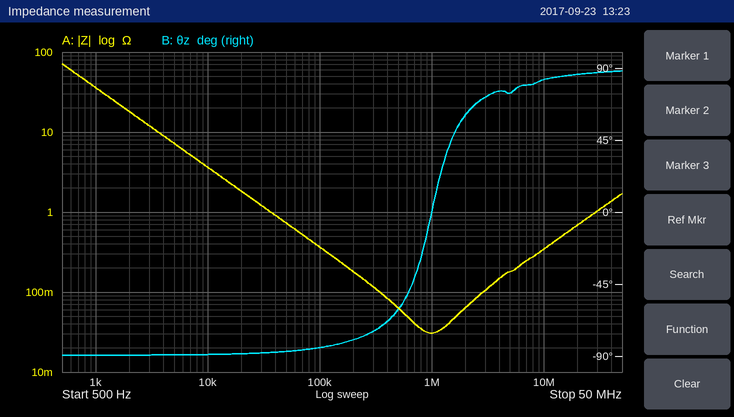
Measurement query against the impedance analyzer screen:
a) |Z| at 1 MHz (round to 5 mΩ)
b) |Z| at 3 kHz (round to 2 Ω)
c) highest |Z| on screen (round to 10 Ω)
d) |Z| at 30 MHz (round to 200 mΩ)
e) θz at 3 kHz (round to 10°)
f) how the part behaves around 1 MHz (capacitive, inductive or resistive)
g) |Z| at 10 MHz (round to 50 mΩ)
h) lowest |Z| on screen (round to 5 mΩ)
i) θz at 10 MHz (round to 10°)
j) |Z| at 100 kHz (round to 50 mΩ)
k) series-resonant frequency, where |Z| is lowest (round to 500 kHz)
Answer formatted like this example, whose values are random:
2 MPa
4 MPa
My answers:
30 mΩ
12 Ω
70 Ω
1.0 Ω
-90°
resistive
350 mΩ
30 mΩ
80°
350 mΩ
1.0 MHz
